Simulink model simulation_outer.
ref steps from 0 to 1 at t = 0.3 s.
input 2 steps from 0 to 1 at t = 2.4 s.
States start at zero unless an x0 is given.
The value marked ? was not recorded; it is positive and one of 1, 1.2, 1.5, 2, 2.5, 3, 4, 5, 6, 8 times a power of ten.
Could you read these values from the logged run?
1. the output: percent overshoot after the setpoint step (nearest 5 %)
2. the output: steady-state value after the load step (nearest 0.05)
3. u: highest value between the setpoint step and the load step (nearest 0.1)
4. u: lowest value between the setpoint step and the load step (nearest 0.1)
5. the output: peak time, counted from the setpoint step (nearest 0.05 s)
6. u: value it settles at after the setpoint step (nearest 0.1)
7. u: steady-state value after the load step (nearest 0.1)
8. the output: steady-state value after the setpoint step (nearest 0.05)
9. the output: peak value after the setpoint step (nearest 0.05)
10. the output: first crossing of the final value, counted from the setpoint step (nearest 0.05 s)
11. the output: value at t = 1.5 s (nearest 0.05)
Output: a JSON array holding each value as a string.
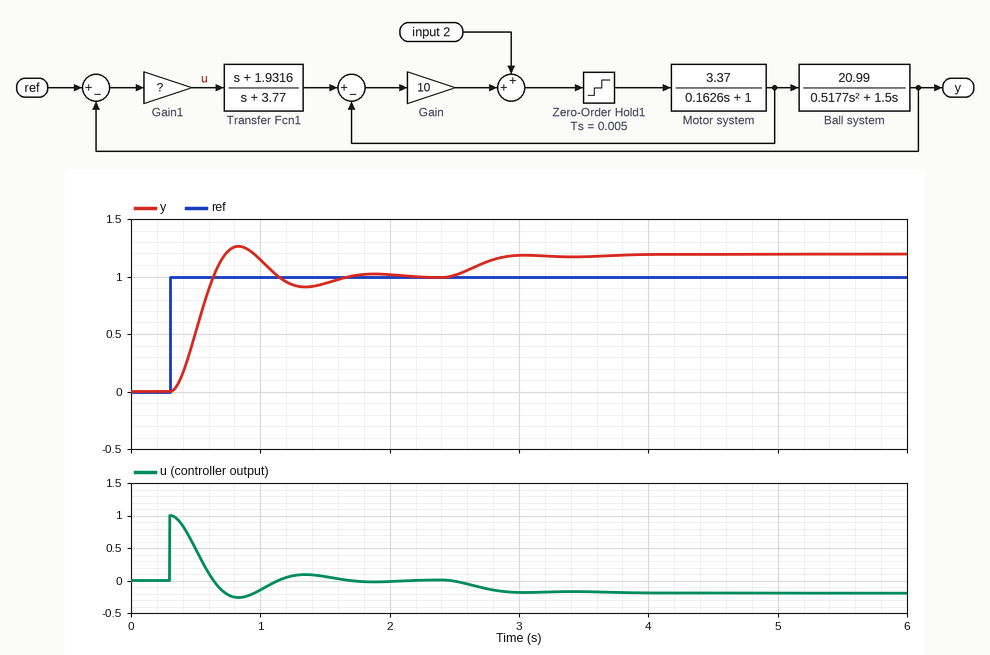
["25 %", "1.20", "1.0", "-0.3", "0.55 s", "0.0", "-0.2", "1.00", "1.25", "0.35 s", "0.95"]
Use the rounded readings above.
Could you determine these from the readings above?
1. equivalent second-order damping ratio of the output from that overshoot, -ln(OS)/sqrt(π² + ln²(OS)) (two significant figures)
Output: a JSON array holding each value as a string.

["0.40"]
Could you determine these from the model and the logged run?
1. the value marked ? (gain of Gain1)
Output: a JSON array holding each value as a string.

["1"]
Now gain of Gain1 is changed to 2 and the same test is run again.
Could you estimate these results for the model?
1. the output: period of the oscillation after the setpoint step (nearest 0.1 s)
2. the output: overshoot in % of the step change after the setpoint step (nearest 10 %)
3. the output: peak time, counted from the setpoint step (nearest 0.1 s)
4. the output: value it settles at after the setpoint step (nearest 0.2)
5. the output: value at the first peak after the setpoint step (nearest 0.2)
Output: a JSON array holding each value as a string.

["0.7 s", "40 %", "0.4 s", "1.0", "1.4"]
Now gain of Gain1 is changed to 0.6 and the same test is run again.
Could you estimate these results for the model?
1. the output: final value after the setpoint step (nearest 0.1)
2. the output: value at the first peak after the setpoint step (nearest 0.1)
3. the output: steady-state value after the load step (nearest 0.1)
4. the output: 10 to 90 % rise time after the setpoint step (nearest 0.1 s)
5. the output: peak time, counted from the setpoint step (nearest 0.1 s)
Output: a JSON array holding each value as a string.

["1.0", "1.1", "1.3", "0.3 s", "0.7 s"]
